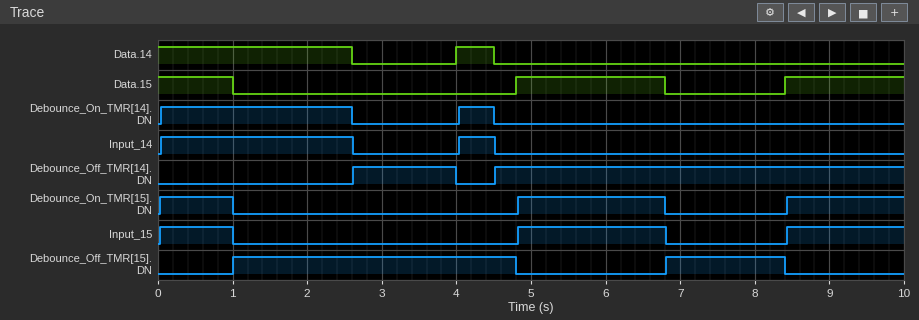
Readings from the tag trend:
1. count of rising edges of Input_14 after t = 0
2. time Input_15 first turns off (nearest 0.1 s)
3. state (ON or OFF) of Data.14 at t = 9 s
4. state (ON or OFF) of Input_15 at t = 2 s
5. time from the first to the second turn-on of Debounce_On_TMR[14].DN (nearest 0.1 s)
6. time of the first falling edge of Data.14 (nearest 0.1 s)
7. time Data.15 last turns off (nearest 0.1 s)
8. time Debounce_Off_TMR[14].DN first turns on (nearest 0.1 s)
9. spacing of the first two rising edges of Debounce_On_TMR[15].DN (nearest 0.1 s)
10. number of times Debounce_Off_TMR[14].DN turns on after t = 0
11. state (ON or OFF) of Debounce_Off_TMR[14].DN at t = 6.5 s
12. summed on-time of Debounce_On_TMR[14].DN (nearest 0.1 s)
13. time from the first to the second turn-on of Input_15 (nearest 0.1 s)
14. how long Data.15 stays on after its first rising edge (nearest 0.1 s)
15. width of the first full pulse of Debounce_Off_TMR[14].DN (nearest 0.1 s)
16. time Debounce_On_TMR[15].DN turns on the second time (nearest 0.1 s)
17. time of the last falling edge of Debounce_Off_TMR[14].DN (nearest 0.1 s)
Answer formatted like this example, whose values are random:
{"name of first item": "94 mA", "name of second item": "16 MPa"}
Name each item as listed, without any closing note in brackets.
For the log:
{"count of rising edges of Input_14 after t = 0": "2", "time Input_15 first turns off": "1.0 s", "state (ON or OFF) of Data.14 at t = 9 s": "OFF", "state (ON or OFF) of Input_15 at t = 2 s": "OFF", "time from the first to the second turn-on of Debounce_On_TMR[14].DN": "4.0 s", "time of the first falling edge of Data.14": "2.6 s", "time Data.15 last turns off": "6.8 s", "time Debounce_Off_TMR[14].DN first turns on": "2.6 s", "spacing of the first two rising edges of Debounce_On_TMR[15].DN": "4.8 s", "number of times Debounce_Off_TMR[14].DN turns on after t = 0": "2", "state (ON or OFF) of Debounce_Off_TMR[14].DN at t = 6.5 s": "ON", "summed on-time of Debounce_On_TMR[14].DN": "3.0 s", "time from the first to the second turn-on of Input_15": "4.8 s", "how long Data.15 stays on after its first rising edge": "2.0 s", "width of the first full pulse of Debounce_Off_TMR[14].DN": "1.4 s", "time Debounce_On_TMR[15].DN turns on the second time": "4.8 s", "time of the last falling edge of Debounce_Off_TMR[14].DN": "4.0 s"}
